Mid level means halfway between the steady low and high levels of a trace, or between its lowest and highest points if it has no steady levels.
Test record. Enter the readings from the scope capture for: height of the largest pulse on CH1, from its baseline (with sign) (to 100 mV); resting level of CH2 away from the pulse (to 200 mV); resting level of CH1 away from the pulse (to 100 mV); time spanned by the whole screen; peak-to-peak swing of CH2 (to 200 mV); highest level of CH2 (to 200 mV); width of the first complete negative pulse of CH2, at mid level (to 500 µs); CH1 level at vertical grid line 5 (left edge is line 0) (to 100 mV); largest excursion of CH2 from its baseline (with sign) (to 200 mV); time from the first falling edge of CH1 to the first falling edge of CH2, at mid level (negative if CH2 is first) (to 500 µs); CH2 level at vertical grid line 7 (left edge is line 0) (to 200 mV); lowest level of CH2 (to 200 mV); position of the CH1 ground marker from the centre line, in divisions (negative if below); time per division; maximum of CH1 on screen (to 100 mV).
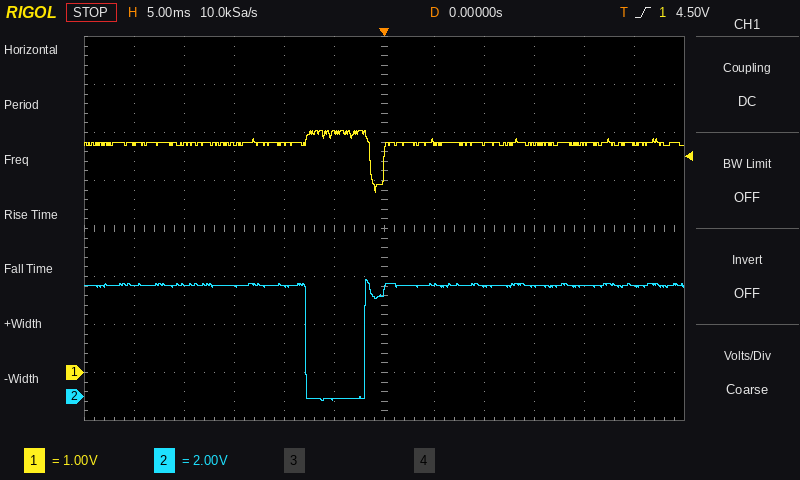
-1.0 V
4.6 V
4.8 V
60 ms
5.0 V
4.8 V
6.0 ms
5.0 V
-4.8 V
-6.5 ms
4.6 V
-200 mV
-3.0 div
5 ms
5.0 V
